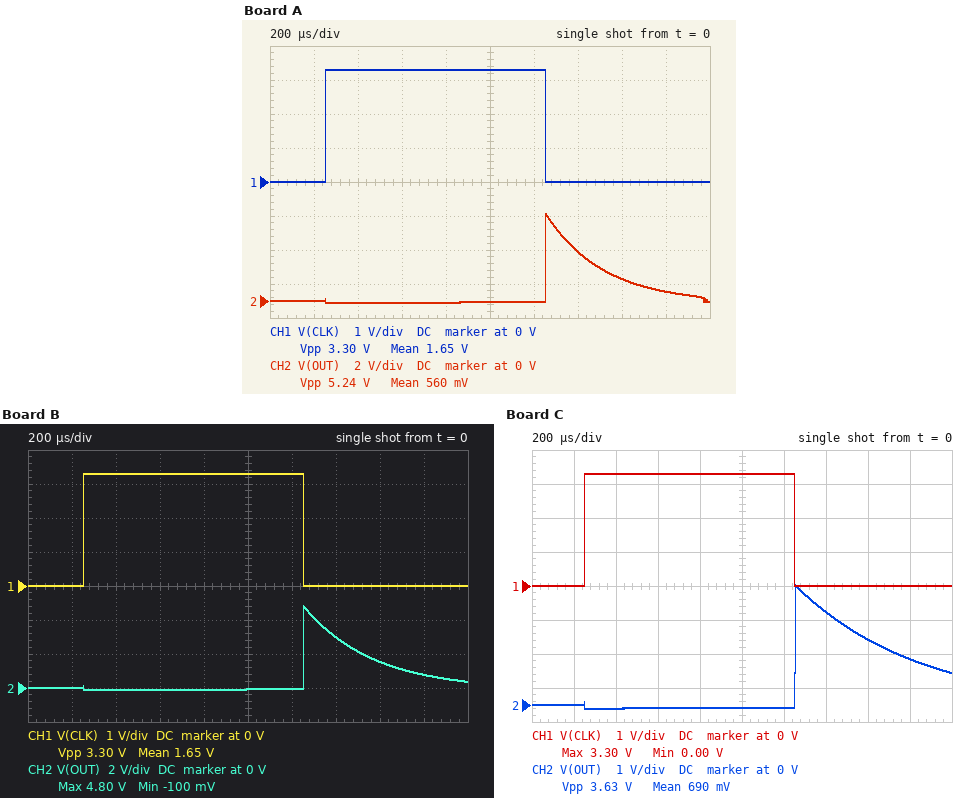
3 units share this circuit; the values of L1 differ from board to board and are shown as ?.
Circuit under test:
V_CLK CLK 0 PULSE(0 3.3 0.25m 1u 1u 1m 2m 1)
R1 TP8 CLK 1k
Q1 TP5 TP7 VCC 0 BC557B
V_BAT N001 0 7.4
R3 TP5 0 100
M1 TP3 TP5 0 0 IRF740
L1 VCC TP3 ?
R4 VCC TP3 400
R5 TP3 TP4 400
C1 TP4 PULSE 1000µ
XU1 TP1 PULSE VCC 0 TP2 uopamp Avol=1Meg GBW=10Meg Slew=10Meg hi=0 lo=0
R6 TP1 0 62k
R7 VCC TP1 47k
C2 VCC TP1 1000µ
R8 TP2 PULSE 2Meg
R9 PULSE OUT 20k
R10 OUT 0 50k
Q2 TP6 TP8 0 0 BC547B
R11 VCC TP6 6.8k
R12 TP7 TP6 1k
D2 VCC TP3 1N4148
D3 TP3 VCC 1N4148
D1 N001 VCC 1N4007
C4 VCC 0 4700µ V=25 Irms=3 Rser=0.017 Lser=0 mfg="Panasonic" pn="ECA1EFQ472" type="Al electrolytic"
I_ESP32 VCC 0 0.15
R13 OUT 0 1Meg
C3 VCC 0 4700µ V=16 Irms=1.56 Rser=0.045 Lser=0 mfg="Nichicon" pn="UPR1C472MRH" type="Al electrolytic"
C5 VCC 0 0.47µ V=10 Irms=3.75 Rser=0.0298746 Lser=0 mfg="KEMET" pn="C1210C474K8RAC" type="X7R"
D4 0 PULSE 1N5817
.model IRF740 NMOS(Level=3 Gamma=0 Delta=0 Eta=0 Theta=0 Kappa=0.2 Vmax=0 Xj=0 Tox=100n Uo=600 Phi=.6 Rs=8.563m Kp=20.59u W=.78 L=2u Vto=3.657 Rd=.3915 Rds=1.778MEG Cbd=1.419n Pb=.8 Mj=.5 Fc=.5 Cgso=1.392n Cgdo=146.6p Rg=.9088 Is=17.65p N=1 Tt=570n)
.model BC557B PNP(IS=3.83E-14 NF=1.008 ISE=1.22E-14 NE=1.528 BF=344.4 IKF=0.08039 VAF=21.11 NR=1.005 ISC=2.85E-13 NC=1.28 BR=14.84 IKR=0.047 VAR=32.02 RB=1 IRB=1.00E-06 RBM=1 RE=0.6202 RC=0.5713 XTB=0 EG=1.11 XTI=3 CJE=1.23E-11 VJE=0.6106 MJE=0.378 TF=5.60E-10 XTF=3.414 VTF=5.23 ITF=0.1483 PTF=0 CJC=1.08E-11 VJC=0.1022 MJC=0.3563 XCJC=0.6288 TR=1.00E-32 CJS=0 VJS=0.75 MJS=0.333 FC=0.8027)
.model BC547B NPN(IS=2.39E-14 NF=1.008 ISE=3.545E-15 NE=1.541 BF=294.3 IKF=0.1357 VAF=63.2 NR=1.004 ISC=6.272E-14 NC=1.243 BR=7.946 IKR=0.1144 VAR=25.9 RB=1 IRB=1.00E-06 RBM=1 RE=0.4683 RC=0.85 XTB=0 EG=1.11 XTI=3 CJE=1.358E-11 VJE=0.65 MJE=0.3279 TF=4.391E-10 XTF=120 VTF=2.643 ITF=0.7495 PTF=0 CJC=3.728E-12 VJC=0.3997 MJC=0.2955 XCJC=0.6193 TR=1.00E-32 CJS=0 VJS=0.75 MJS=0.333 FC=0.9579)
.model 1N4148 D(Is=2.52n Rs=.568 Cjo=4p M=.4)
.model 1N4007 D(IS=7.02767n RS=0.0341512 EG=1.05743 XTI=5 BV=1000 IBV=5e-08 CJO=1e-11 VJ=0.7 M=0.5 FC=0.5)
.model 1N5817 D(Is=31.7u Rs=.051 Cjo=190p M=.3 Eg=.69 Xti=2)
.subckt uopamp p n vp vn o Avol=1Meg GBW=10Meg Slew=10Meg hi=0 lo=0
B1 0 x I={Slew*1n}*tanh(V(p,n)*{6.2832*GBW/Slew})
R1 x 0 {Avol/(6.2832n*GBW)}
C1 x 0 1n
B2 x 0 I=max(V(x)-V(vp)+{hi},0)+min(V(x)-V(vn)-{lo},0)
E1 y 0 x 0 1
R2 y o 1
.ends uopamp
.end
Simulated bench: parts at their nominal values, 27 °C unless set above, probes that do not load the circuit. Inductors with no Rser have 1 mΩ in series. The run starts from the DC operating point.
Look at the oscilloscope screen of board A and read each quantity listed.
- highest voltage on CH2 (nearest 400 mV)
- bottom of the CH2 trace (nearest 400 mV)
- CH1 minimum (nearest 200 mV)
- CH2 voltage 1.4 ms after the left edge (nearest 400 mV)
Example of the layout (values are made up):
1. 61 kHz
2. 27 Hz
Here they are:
1. 5.2 V
2. 0 V
3. 0 V
4. 2.8 V
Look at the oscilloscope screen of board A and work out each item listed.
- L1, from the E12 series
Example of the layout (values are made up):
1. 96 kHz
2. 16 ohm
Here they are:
1. 150 µH
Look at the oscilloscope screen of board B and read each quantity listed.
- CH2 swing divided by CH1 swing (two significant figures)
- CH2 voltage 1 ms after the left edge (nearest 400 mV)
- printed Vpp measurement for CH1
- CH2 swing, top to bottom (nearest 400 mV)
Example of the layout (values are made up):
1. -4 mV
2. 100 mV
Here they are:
1. 1.5
2. 0 V
3. 3.30 V
4. 4.8 V
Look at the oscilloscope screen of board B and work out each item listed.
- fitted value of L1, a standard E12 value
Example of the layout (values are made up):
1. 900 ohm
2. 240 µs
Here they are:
1. 180 µH
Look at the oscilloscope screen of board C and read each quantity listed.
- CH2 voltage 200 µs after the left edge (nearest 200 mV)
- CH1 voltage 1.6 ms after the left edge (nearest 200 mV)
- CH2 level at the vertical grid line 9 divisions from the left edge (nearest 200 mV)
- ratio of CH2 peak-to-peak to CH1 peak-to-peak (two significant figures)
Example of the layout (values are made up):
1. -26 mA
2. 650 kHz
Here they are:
1. 0 V
2. 0 V
3. 1.4 V
4. 1.1
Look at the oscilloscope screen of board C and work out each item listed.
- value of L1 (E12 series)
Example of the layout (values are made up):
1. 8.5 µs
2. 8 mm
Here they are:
1. 330 µH
